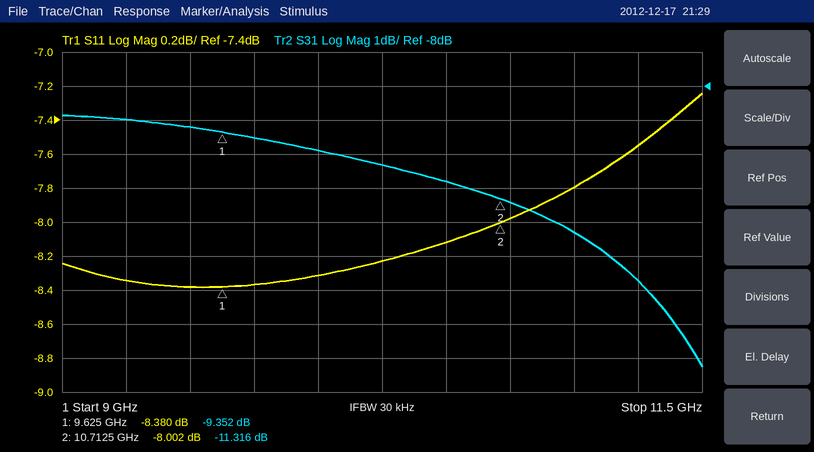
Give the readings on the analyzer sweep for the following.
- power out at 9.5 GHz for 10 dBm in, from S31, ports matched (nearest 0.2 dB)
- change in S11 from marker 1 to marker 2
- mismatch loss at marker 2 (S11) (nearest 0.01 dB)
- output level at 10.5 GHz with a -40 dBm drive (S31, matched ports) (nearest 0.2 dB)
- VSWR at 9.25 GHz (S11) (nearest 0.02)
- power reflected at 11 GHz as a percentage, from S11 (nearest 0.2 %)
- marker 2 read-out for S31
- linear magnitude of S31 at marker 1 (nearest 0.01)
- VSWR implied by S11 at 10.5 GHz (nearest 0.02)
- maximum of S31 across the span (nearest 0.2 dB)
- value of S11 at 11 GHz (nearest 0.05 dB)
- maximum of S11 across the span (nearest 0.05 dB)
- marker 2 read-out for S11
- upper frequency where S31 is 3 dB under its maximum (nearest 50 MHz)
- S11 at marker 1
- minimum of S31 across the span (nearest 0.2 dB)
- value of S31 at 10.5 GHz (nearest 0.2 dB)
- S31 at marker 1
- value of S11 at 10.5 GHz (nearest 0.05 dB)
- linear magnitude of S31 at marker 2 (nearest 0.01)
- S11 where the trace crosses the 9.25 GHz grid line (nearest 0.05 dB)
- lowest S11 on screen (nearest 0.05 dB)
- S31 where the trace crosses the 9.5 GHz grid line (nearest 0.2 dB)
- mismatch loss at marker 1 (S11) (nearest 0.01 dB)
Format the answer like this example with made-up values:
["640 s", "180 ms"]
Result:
["0.8 dBm", "0.378 dB", "0.75 dB", "-50.8 dBm", "2.24", "16.6 %", "-11.316 dB", "0.34", "2.30", "-8.8 dB", "-7.80 dB", "-7.25 dB", "-8.002 dB", "10.90 GHz", "-8.380 dB", "-16.2 dB", "-10.8 dB", "-9.352 dB", "-8.10 dB", "0.27", "-8.35 dB", "-8.40 dB", "-9.2 dB", "0.68 dB"]
